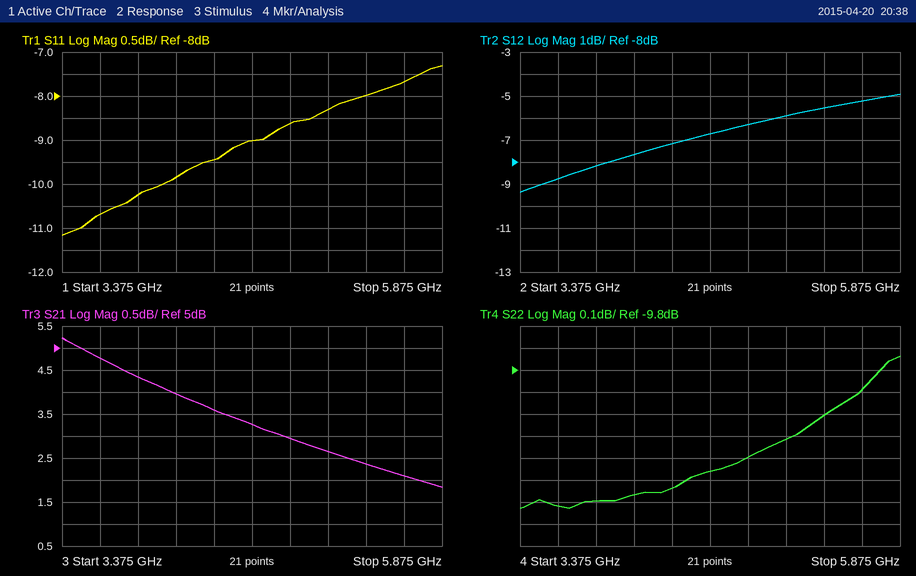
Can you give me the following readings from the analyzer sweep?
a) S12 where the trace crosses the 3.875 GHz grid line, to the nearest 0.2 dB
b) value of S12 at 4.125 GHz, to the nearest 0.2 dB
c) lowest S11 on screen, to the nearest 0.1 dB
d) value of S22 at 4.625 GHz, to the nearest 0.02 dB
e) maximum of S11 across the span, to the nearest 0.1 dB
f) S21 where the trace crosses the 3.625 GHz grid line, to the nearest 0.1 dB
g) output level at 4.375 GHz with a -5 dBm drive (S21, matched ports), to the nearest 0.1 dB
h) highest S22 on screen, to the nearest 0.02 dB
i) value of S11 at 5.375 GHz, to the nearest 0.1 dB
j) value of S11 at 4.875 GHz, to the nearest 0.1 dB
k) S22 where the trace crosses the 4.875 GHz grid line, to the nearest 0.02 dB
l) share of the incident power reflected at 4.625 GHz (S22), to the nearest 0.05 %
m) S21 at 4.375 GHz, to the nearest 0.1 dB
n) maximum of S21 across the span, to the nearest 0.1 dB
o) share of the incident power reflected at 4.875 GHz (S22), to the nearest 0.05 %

-8.2 dB
-7.6 dB
-11.2 dB
-10.26 dB
-7.3 dB
4.8 dB
-1.4 dBm
-9.74 dB
-8.0 dB
-8.6 dB
-10.20 dB
9.40 %
3.6 dB
5.2 dB
9.55 %
